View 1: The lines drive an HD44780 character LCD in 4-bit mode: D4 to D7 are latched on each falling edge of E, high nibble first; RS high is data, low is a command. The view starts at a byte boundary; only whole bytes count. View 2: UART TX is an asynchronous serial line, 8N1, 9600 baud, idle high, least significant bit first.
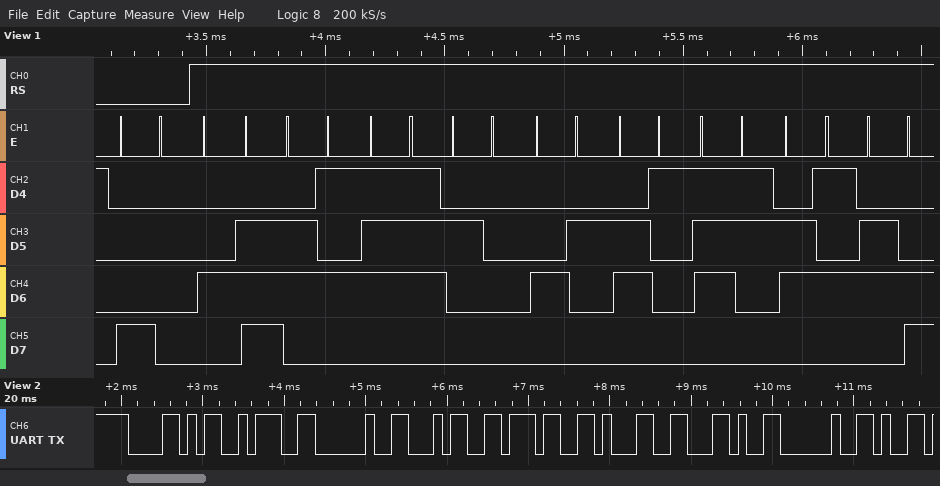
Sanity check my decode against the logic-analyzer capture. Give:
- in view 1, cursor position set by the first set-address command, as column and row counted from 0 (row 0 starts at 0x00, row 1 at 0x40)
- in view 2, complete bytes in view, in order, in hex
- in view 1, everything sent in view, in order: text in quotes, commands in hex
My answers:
column 0, row 0
0x58 0x3A 0x20 0x34 0x37 0x31 0x2C 0x20
0x80 "New Basel"
